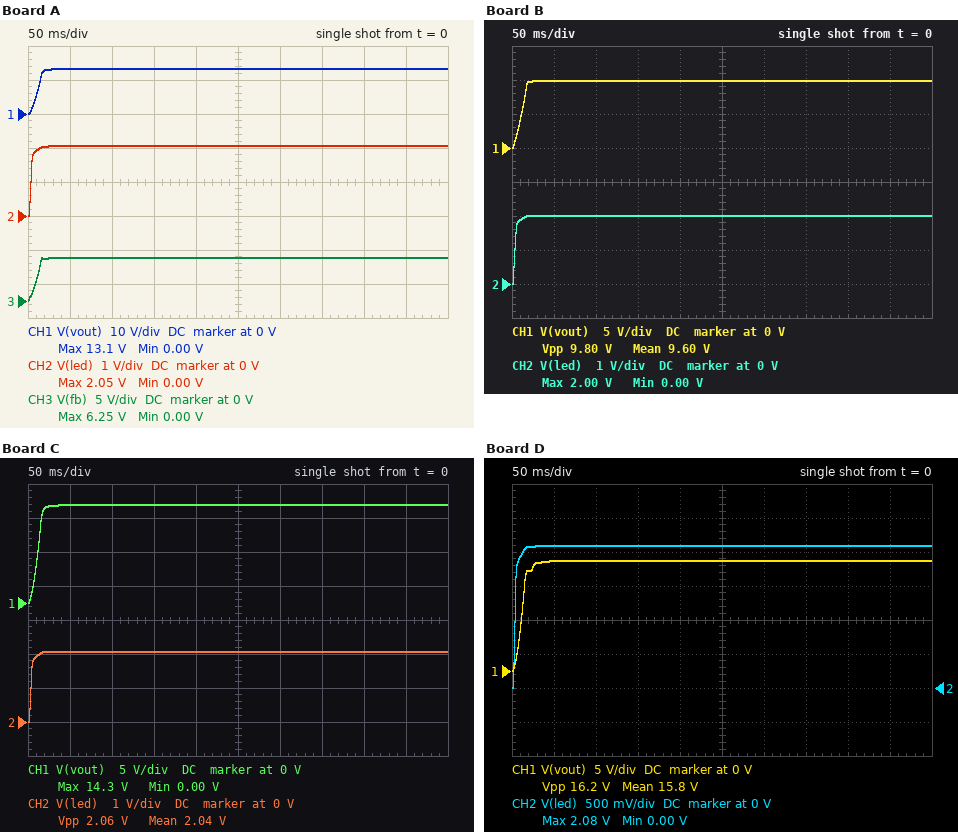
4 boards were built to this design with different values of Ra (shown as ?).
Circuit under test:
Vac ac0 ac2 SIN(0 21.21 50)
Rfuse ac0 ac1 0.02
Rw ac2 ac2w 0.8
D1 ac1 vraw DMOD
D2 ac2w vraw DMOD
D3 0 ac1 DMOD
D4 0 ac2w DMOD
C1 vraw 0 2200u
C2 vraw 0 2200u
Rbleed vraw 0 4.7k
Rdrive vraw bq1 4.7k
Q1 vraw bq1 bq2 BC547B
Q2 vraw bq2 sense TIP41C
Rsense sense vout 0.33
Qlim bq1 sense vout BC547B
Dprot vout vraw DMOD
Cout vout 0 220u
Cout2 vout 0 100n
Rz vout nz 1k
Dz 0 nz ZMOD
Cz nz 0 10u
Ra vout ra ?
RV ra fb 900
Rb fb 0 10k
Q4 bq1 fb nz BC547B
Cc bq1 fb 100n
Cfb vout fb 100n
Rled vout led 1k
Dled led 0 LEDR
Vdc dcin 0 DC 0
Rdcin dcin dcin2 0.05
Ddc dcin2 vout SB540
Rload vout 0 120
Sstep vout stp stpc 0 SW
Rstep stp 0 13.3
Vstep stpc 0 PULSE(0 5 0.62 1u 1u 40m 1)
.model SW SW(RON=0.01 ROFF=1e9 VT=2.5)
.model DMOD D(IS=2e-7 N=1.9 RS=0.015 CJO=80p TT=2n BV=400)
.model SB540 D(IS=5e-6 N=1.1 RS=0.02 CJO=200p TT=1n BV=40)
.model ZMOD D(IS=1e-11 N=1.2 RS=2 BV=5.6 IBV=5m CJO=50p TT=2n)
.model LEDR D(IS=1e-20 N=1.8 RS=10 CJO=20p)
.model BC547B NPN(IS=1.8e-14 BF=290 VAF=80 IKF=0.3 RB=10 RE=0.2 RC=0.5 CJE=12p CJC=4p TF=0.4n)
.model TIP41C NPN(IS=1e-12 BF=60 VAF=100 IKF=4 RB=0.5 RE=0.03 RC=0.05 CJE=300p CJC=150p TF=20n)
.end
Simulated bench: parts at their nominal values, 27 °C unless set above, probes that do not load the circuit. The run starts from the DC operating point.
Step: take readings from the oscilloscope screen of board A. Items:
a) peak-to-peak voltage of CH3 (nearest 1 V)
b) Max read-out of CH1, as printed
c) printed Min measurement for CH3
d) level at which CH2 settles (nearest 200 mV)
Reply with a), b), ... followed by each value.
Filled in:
a) 6 V
b) 13.1 V
c) 0.00 V
d) 2.0 V
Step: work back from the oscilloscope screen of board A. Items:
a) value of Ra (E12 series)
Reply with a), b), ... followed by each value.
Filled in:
a) 10 kΩ
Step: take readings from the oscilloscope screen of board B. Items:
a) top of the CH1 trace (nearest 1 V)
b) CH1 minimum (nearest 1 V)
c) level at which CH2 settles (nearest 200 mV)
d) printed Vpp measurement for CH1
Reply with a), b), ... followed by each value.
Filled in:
a) 10 V
b) 0 V
c) 2.0 V
d) 9.80 V
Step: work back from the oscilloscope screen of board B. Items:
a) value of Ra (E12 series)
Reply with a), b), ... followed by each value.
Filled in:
a) 4.7 kΩ
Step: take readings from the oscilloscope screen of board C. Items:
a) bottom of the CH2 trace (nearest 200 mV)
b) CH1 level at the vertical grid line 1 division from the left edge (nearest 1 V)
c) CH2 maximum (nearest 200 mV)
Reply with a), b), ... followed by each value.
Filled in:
a) 0 V
b) 14 V
c) 2.0 V
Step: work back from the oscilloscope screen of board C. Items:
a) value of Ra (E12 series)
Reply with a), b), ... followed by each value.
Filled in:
a) 12 kΩ
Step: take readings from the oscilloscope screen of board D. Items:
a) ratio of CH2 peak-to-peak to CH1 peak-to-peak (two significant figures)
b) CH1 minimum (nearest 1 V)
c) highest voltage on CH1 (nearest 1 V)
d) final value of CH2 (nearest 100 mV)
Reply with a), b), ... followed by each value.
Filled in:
a) 0.13
b) 0 V
c) 16 V
d) 2.1 V
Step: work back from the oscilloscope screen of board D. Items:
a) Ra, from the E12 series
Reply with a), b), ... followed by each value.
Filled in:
a) 15 kΩ
